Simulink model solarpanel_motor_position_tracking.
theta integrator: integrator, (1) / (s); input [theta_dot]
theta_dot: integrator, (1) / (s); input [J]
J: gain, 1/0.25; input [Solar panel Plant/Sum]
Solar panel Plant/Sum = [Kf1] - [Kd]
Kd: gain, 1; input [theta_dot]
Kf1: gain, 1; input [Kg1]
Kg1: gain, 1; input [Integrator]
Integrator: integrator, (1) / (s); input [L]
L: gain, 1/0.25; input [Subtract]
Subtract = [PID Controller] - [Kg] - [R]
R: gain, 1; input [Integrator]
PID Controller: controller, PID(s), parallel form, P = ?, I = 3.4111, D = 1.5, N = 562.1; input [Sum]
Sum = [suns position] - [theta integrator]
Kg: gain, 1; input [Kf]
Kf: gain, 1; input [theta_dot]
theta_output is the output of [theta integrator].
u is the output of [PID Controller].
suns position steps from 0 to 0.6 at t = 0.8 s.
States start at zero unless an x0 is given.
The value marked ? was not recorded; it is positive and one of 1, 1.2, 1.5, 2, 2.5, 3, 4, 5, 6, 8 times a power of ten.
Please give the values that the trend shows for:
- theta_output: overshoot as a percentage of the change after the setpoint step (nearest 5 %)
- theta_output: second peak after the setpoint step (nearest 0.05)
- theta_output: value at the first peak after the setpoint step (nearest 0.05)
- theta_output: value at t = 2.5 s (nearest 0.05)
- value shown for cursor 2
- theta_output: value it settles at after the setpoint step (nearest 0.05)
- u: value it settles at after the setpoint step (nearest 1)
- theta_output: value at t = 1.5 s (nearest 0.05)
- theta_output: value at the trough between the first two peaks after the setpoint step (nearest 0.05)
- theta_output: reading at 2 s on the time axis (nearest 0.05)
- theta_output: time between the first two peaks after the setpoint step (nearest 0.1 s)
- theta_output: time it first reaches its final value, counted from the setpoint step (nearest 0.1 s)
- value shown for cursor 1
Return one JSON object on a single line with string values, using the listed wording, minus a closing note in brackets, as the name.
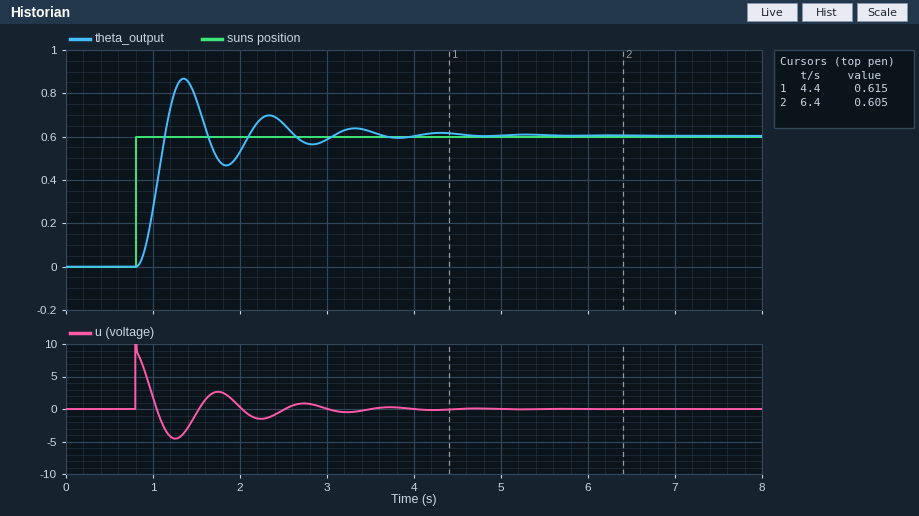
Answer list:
{"theta_output: overshoot as a percentage of the change after the setpoint step": "45 %", "theta_output: second peak after the setpoint step": "0.70", "theta_output: value at the first peak after the setpoint step": "0.85", "theta_output: value at t = 2.5 s": "0.65", "value shown for cursor 2": "0.605", "theta_output: value it settles at after the setpoint step": "0.60", "u: value it settles at after the setpoint step": "0", "theta_output: value at t = 1.5 s": "0.75", "theta_output: value at the trough between the first two peaks after the setpoint step": "0.45", "theta_output: reading at 2 s on the time axis": "0.55", "theta_output: time between the first two peaks after the setpoint step": "1.0 s", "theta_output: time it first reaches its final value, counted from the setpoint step": "0.3 s", "value shown for cursor 1": "0.615"}
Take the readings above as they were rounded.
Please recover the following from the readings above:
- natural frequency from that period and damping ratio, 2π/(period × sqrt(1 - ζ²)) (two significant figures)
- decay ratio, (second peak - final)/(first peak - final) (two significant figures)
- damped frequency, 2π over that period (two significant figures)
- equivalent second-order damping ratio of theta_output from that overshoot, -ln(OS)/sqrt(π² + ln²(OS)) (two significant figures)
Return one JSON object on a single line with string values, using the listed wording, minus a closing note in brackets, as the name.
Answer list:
{"natural frequency from that period and damping ratio, 2π/(period × sqrt(1 - ζ²))": "6.5 rad/s", "decay ratio, (second peak - final)/(first peak - final)": "0.40", "damped frequency, 2π over that period": "6.3 rad/s", "equivalent second-order damping ratio of theta_output from that overshoot, -ln(OS)/sqrt(π² + ln²(OS))": "0.25"}
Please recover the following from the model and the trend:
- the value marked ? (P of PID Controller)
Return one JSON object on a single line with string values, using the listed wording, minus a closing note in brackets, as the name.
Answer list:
{"the value marked ?": "15"}
